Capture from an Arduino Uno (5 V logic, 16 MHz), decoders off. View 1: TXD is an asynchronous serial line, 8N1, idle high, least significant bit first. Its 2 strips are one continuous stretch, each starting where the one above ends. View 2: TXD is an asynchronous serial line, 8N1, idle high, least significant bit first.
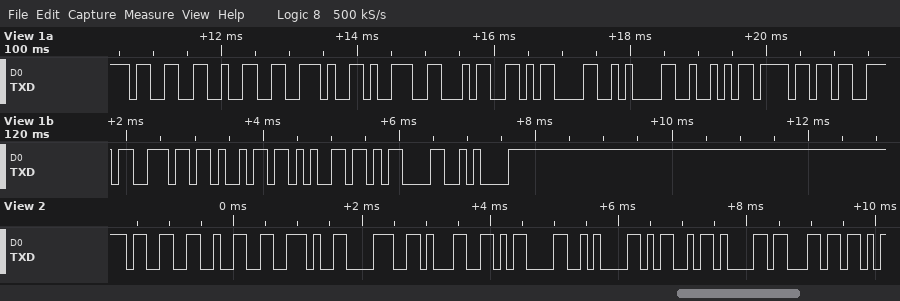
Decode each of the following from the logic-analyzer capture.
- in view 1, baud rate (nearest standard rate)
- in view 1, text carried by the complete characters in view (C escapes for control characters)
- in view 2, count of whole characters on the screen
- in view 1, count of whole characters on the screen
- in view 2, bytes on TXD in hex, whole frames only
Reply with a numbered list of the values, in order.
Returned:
1. 9600 baud
2. "32.94\r\nRosnie\r\n"
3. 10
4. 15
5. 0x33 0x32 0x2E 0x38 0x31 0x0D 0x0A 0x4D 0x61 0x6C
